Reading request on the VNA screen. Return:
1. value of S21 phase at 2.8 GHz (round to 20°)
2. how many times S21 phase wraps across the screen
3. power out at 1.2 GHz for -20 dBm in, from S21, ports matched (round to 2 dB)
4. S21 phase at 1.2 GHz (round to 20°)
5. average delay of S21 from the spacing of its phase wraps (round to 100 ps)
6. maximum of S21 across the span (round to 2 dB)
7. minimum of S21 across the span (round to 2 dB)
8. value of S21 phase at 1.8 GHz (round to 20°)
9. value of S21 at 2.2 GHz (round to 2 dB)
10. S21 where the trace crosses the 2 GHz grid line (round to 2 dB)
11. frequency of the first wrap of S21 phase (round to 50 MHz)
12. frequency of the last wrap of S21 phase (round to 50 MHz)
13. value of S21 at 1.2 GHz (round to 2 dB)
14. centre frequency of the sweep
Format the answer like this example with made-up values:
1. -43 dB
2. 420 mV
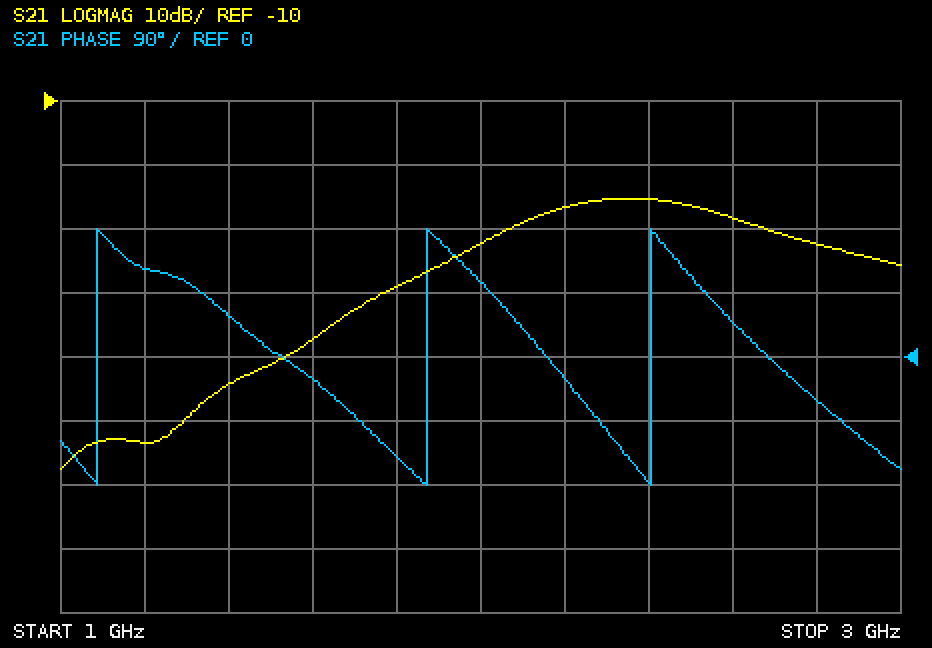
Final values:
1. -60°
2. 3
3. -84 dBm
4. 120°
5. 1.5 ns
6. -26 dB
7. -68 dB
8. -140°
9. -26 dB
10. -32 dB
11. 1.10 GHz
12. 2.40 GHz
13. -64 dB
14. 2 GHz
